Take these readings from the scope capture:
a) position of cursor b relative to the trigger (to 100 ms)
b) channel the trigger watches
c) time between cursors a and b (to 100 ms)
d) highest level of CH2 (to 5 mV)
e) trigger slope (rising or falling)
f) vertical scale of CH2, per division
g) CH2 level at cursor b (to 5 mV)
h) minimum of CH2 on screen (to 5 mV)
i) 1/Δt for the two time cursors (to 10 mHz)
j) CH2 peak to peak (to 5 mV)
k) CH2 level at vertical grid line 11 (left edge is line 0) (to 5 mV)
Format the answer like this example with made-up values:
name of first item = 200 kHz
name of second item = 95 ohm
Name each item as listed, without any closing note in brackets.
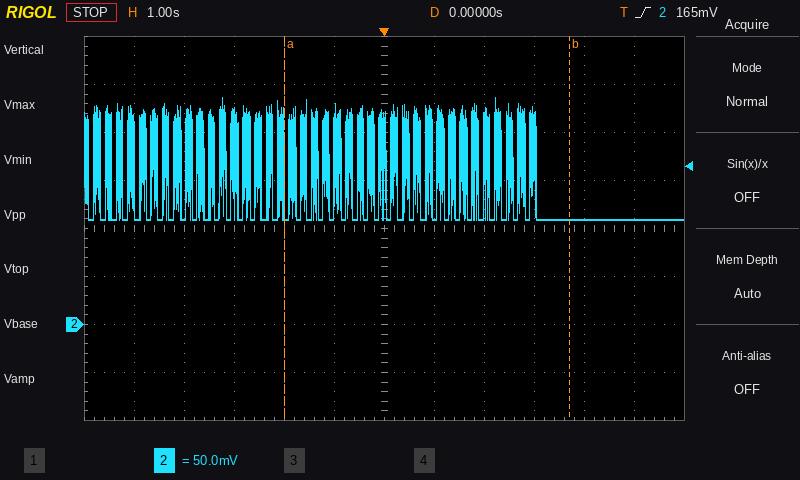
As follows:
position of cursor b relative to the trigger = +3.7 s
channel the trigger watches = CH2
time between cursors a and b = 5.7 s
highest level of CH2 = 235 mV
trigger slope = rising
vertical scale of CH2, per division = 50 mV
CH2 level at cursor b = 110 mV
minimum of CH2 on screen = 110 mV
1/Δt for the two time cursors = 180 mHz
CH2 peak to peak = 125 mV
CH2 level at vertical grid line 11 (left edge is line 0) = 110 mV
